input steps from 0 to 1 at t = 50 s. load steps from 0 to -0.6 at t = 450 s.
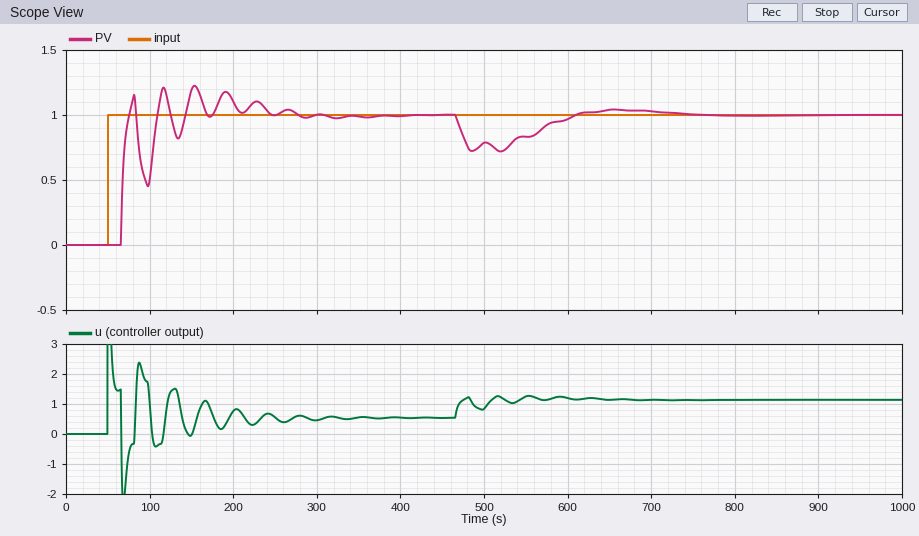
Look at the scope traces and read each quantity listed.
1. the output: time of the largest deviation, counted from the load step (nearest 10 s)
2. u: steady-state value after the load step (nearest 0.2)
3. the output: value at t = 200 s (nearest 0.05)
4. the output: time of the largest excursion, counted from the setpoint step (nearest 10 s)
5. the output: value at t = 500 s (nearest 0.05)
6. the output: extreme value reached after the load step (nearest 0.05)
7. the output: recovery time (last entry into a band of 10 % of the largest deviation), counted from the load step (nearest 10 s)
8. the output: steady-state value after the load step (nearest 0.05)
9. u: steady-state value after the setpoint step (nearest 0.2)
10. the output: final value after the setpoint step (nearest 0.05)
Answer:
70 s
1.2
1.10
100 s
0.80
0.70
250 s
1.00
0.6
1.00
